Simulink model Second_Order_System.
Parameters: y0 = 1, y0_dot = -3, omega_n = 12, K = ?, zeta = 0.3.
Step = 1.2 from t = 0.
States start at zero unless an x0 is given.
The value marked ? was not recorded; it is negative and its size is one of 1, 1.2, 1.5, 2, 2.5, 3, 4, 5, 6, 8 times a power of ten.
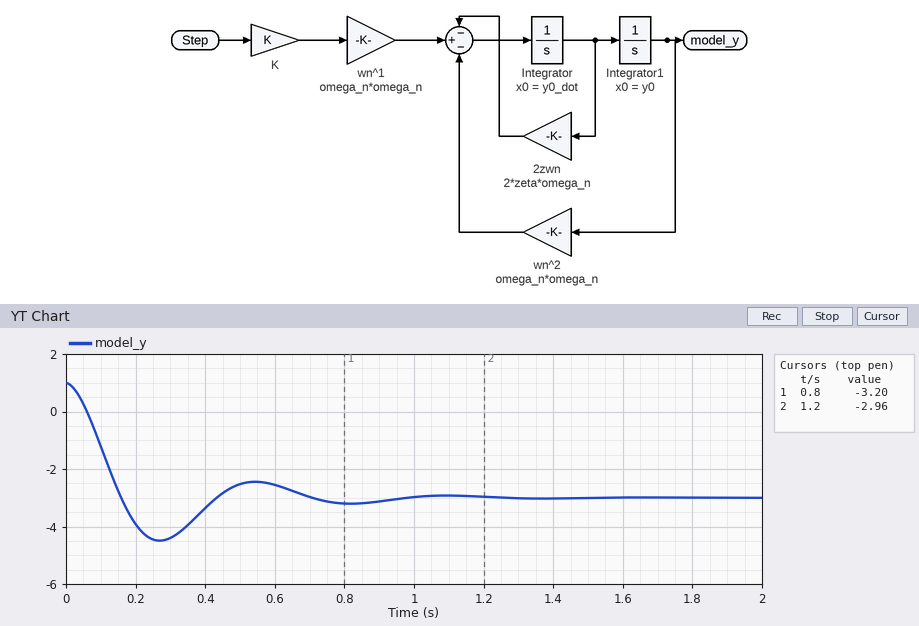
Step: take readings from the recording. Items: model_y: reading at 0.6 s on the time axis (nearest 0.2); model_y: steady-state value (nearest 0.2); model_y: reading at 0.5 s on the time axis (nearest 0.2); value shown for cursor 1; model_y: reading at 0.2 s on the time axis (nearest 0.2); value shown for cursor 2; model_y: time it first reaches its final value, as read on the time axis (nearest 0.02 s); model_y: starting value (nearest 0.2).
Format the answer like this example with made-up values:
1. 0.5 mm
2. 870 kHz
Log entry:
1. -2.6
2. -3.0
3. -2.6
4. -3.20
5. -4.0
6. -2.96
7. 0.16 s
8. 1.0
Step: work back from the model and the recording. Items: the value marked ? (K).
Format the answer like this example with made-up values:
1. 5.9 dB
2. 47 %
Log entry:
1. -2.5
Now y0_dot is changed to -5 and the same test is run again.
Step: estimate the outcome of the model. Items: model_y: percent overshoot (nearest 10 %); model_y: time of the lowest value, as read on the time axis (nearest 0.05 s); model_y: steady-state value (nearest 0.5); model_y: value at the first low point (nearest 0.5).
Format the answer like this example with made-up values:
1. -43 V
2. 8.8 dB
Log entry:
1. 40 %
2. 0.25 s
3. -3.0
4. -4.5
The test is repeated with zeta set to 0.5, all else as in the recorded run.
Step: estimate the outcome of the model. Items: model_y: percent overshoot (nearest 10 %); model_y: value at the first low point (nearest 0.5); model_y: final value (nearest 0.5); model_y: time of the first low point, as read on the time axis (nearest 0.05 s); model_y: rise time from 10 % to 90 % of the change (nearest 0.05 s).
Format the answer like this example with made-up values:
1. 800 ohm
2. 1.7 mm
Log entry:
1. 20 %
2. -3.5
3. -3.0
4. 0.30 s
5. 0.15 s
